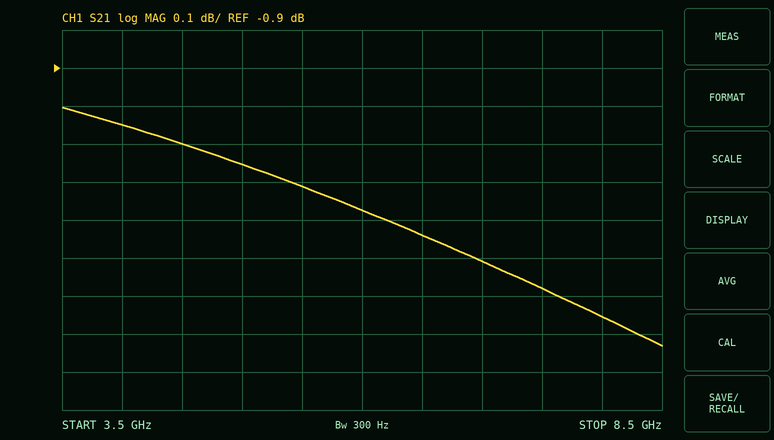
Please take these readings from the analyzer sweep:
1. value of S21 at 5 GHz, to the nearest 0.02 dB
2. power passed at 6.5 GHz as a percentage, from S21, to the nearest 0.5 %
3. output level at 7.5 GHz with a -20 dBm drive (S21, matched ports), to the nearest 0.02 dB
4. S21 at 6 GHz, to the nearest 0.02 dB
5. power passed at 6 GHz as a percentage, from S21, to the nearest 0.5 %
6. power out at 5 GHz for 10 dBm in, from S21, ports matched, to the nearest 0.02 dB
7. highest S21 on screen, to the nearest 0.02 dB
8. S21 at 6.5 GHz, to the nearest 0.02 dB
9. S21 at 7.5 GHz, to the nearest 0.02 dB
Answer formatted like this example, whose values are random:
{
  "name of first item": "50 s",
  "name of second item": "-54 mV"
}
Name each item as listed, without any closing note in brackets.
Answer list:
{
  "value of S21 at 5 GHz, to the nearest 0.02 dB": "-1.16 dB",
  "power passed at 6.5 GHz as a percentage, from S21, to the nearest 0.5 %": "73.5 %",
  "output level at 7.5 GHz with a -20 dBm drive (S21, matched ports), to the nearest 0.02 dB": "-21.48 dBm",
  "S21 at 6 GHz, to the nearest 0.02 dB": "-1.28 dB",
  "power passed at 6 GHz as a percentage, from S21, to the nearest 0.5 %": "74.5 %",
  "power out at 5 GHz for 10 dBm in, from S21, ports matched, to the nearest 0.02 dB": "8.84 dBm",
  "highest S21 on screen, to the nearest 0.02 dB": "-1.00 dB",
  "S21 at 6.5 GHz, to the nearest 0.02 dB": "-1.34 dB",
  "S21 at 7.5 GHz, to the nearest 0.02 dB": "-1.48 dB"
}
